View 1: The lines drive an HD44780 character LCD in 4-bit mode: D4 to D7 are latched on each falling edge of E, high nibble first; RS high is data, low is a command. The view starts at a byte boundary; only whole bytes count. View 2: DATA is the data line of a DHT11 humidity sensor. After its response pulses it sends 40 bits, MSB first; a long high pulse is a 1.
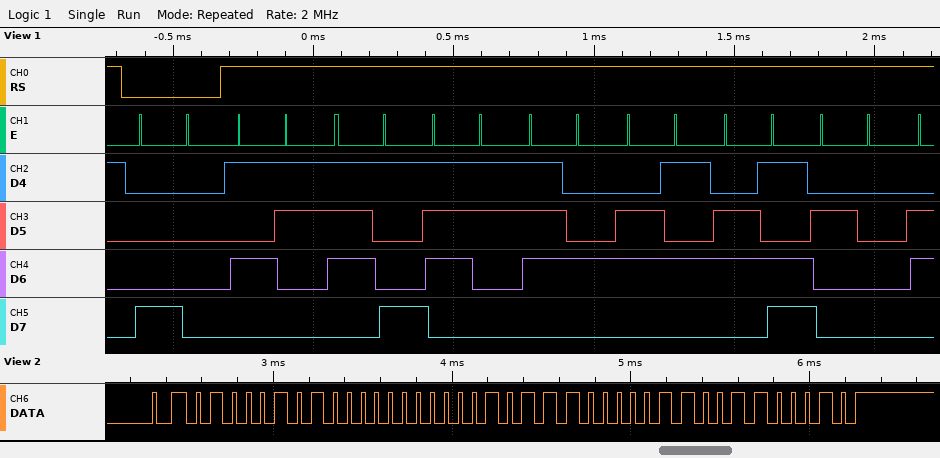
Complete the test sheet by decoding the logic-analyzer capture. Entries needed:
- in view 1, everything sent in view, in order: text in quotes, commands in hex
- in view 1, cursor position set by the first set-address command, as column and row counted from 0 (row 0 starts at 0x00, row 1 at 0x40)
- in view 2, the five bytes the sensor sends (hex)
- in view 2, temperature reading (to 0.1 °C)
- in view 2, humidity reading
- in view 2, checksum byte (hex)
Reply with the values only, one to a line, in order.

0x80 "System "
column 0, row 0
45 00 17 06 62
23.6 °C
69 %
0x62
